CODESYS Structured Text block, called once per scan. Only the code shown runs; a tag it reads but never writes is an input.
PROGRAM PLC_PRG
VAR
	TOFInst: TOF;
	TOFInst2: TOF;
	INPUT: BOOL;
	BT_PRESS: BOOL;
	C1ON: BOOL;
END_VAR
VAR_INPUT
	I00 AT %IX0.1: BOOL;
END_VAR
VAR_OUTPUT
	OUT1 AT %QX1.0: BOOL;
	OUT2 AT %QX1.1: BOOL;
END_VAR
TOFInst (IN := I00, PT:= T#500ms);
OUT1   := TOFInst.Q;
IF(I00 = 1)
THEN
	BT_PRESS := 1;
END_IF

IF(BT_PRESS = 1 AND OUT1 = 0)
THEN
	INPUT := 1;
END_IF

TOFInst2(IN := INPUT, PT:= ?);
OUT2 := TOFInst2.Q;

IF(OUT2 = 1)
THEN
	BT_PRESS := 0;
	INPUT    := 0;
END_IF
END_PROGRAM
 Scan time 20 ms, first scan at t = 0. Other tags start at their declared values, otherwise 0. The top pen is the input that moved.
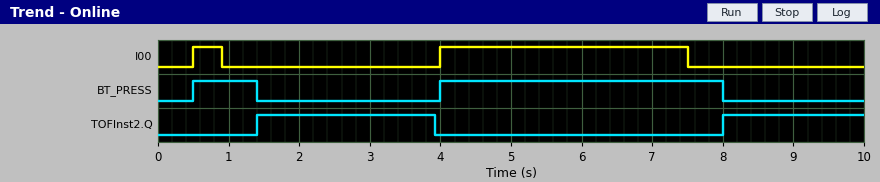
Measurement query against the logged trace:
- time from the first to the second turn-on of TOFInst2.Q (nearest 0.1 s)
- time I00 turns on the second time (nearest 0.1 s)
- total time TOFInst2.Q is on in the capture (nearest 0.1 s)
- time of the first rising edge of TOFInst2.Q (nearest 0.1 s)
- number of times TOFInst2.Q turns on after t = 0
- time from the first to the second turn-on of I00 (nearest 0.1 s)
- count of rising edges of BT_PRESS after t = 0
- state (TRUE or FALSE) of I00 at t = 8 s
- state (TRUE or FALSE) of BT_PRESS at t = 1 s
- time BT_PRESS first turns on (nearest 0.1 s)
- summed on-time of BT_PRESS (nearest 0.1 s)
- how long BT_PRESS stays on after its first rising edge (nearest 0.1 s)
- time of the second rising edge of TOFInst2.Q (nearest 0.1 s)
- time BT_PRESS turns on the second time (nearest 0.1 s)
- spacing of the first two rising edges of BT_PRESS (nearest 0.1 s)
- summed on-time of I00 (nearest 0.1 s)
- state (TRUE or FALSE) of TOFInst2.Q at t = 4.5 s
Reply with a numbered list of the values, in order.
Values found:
1. 6.6 s
2. 4.0 s
3. 4.5 s
4. 1.4 s
5. 2
6. 3.5 s
7. 2
8. FALSE
9. TRUE
10. 0.5 s
11. 4.9 s
12. 0.9 s
13. 8.0 s
14. 4.0 s
15. 3.5 s
16. 3.9 s
17. FALSE
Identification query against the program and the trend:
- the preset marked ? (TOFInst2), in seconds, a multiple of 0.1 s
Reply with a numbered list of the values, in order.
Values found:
1. 2.5 s
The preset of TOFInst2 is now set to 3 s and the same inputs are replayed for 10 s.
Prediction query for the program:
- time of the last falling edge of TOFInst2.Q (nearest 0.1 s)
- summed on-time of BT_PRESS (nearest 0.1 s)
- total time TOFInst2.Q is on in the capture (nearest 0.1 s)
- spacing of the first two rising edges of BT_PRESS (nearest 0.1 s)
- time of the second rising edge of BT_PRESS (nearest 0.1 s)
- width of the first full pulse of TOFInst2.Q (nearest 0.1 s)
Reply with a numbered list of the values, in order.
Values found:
1. 4.4 s
2. 4.5 s
3. 5.0 s
4. 3.9 s
5. 4.4 s
6. 3.0 s
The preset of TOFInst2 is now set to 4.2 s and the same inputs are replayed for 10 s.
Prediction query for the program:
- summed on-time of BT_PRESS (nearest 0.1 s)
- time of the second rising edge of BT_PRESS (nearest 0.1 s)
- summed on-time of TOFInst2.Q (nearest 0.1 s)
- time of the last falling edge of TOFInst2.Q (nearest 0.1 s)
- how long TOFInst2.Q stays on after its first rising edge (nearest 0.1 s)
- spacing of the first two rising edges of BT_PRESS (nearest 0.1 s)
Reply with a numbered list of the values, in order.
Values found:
1. 3.3 s
2. 5.6 s
3. 6.2 s
4. 5.6 s
5. 4.2 s
6. 5.1 s
